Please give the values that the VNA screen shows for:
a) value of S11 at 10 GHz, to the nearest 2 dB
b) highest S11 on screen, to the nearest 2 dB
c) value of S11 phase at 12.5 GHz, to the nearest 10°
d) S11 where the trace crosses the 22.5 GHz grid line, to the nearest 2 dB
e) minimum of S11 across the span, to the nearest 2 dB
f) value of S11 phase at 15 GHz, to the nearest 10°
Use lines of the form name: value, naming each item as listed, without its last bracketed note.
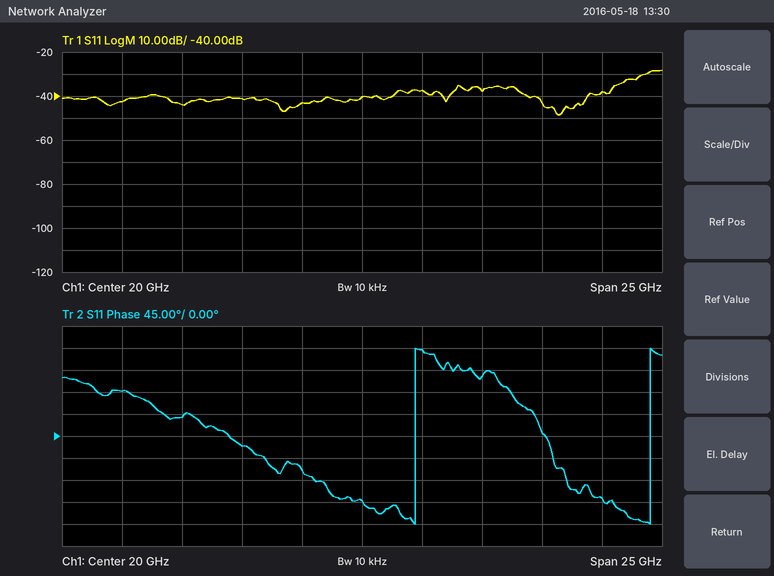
value of S11 at 10 GHz, to the nearest 2 dB: -42 dB
highest S11 on screen, to the nearest 2 dB: -28 dB
value of S11 phase at 12.5 GHz, to the nearest 10°: 40°
S11 where the trace crosses the 22.5 GHz grid line, to the nearest 2 dB: -38 dB
minimum of S11 across the span, to the nearest 2 dB: -48 dB
value of S11 phase at 15 GHz, to the nearest 10°: -20°
